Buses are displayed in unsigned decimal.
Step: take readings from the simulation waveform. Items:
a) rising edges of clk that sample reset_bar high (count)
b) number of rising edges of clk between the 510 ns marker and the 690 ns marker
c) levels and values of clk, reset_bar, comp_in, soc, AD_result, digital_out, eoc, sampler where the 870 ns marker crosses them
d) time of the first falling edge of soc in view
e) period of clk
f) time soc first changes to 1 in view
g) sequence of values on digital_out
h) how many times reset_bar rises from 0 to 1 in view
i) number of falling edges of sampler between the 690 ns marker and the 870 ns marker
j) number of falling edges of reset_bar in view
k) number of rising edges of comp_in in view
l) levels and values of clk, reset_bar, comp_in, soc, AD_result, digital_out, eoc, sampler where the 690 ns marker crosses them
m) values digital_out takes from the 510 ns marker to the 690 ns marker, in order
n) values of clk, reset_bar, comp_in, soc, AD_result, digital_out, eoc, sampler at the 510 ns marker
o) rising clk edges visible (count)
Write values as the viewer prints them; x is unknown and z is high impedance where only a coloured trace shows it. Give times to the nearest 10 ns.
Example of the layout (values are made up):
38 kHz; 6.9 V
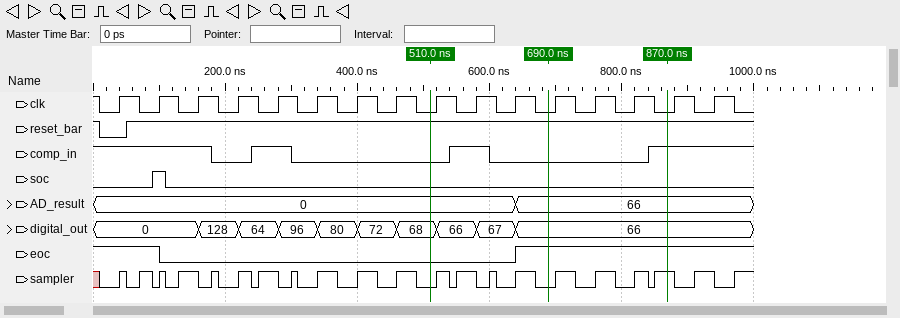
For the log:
15; 3; clk=0, reset_bar=1, comp_in=1, soc=0, AD_result=66, digital_out=66, eoc=1, sampler=1; 110 ns; 60 ns; 90 ns; 0, 128, 64, 96, 80, 72, 68, 66, 67, 66; 1; 3; 1; 3; clk=0, reset_bar=1, comp_in=0, soc=0, AD_result=66, digital_out=66, eoc=1, sampler=0; 68, 66, 67, 66; clk=0, reset_bar=1, comp_in=0, soc=0, AD_result=0, digital_out=68, eoc=0, sampler=0; 16
